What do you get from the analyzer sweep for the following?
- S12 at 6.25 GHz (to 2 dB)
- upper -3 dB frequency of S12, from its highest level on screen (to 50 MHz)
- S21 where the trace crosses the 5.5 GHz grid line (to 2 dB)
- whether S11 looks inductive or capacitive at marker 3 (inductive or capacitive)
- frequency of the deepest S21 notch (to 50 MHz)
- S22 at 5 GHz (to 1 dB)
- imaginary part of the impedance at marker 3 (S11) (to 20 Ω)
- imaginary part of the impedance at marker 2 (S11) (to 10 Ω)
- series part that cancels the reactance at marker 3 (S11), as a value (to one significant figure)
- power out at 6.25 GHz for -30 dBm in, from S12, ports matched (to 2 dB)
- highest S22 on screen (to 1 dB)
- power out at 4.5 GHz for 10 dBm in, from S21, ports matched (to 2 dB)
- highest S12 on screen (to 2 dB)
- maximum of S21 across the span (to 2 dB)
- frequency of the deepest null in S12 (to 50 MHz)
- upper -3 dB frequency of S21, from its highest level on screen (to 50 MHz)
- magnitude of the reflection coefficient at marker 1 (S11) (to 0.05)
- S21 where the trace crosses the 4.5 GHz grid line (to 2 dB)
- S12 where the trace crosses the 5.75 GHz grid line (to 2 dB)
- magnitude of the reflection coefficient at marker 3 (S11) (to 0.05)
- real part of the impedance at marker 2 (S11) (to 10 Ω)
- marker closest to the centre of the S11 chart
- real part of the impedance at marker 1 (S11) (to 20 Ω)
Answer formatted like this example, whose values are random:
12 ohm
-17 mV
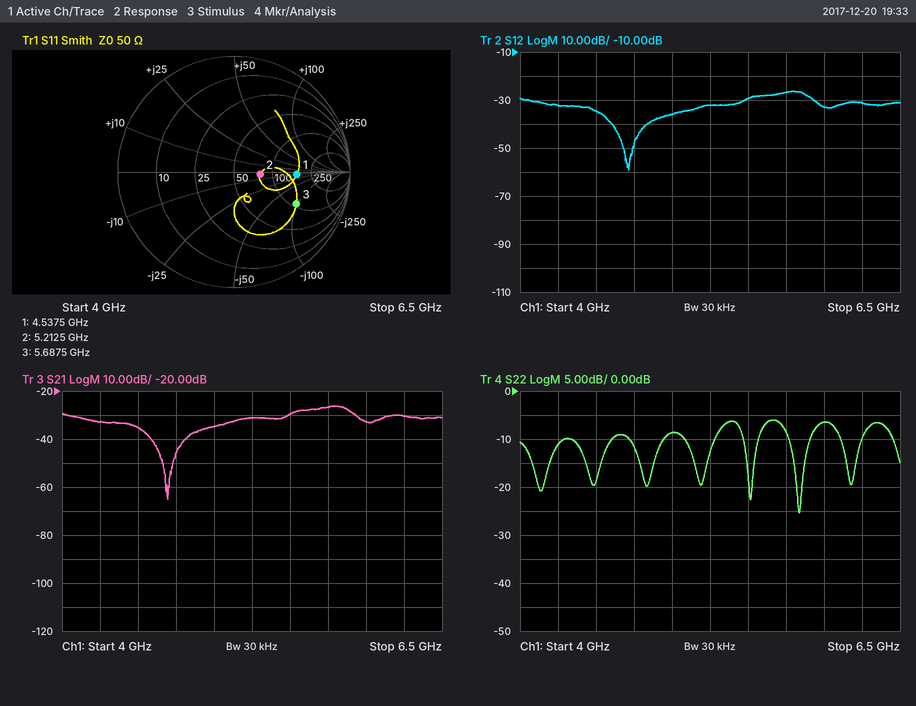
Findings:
-32 dB
5.90 GHz
-30 dB
capacitive
4.70 GHz
-9 dB
-100 Ω
0 Ω
3 nH
-62 dBm
-6 dB
-26 dBm
-26 dB
-26 dB
4.70 GHz
5.90 GHz
0.55
-36 dB
-26 dB
0.60
80 Ω
marker 2
160 Ω
